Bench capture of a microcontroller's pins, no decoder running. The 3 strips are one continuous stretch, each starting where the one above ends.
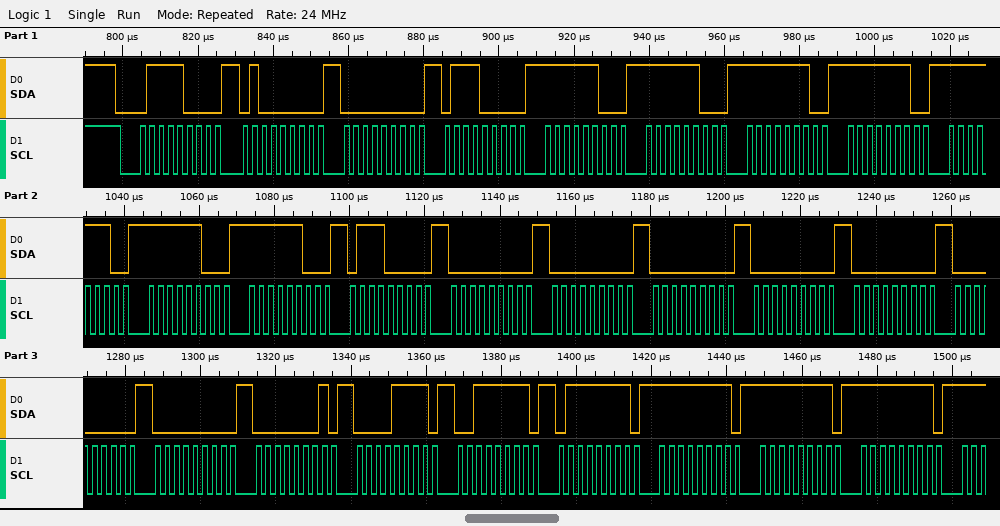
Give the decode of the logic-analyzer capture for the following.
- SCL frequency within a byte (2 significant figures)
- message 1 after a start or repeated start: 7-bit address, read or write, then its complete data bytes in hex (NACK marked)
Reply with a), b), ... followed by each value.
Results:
a) 400 kHz
b) 0x3C write: 40 00 70 FC FC FE FE FE FC FC 70 00 00 00 00 00 00 00 01 0F 3F 7F FF FF FF
